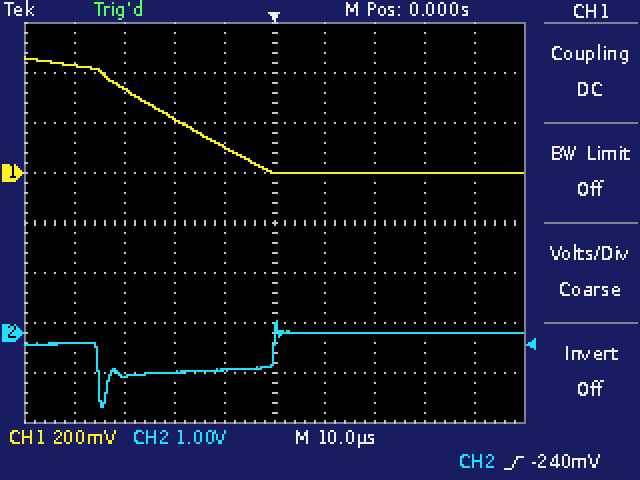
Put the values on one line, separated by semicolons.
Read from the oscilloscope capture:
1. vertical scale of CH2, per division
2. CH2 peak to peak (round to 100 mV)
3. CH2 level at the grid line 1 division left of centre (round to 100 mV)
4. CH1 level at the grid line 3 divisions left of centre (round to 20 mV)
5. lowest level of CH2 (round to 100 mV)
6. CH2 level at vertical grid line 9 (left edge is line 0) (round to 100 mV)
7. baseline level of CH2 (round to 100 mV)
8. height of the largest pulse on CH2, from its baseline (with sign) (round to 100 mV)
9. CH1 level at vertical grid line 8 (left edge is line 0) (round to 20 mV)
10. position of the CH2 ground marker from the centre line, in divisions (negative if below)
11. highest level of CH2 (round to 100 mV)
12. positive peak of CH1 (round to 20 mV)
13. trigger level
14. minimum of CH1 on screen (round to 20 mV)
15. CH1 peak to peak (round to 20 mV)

1 V; 1.7 V; -700 mV; 340 mV; -1.5 V; 0.0 V; 0.0 V; -1.5 V; 0 mV; -2.2 div; 200 mV; 460 mV; -240 mV; 0 mV; 460 mV
